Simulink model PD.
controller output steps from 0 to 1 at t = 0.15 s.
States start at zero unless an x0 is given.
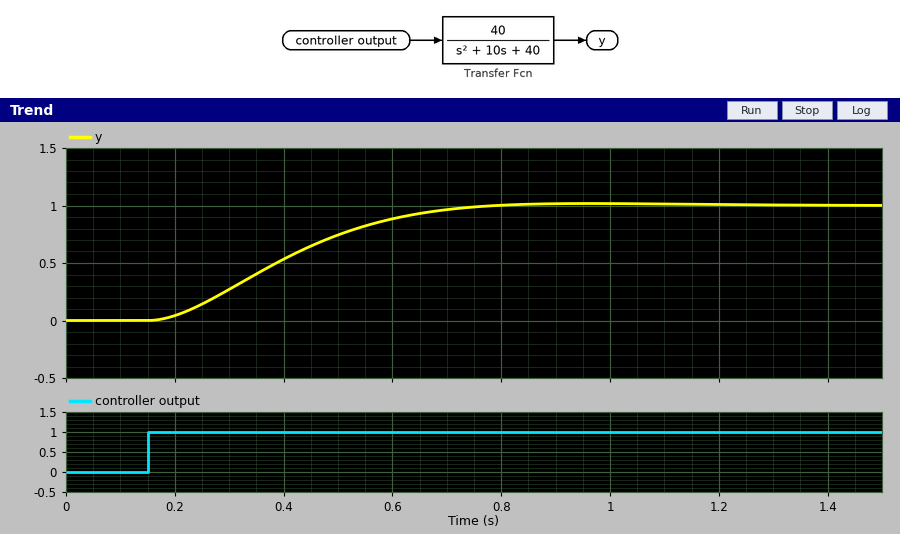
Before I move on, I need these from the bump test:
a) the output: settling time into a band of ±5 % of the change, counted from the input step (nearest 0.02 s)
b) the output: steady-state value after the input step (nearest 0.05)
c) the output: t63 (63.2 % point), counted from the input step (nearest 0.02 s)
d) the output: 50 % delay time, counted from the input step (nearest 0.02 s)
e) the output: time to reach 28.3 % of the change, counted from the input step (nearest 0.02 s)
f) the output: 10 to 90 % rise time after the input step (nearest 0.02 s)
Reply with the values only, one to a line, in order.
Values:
0.52 s
1.00
0.30 s
0.24 s
0.16 s
0.38 s
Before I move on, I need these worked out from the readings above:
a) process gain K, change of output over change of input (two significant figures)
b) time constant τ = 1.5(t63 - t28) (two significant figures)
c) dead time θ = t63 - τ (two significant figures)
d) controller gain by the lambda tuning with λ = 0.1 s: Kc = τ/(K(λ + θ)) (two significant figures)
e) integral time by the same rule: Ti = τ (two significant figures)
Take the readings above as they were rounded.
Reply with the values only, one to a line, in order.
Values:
1.0
0.21 s
0.090 s
1.1
0.21 s
